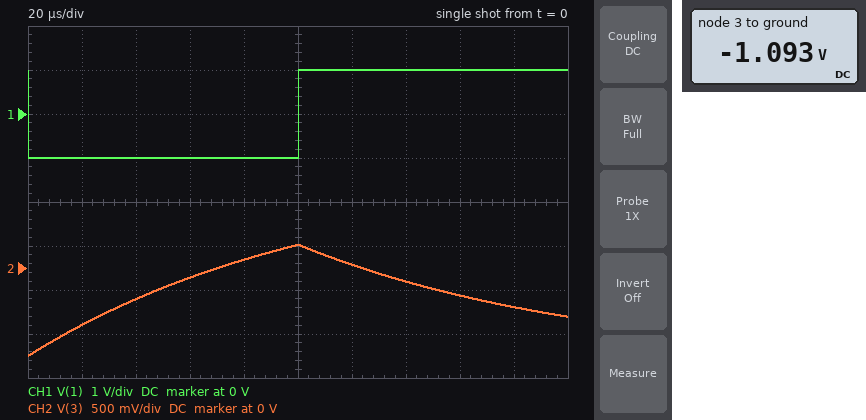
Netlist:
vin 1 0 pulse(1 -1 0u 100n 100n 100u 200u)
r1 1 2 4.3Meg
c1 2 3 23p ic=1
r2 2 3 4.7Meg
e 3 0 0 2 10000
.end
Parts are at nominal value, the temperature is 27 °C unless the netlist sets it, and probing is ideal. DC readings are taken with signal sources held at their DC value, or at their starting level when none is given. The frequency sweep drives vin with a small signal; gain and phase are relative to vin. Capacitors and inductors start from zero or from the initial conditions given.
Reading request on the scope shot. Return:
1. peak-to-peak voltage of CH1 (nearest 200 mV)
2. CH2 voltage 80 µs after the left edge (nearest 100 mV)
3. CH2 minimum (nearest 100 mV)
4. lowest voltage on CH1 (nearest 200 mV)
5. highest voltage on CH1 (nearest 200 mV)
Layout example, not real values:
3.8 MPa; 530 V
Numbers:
2.0 V; 100 mV; -1.0 V; -1.0 V; 1.0 V
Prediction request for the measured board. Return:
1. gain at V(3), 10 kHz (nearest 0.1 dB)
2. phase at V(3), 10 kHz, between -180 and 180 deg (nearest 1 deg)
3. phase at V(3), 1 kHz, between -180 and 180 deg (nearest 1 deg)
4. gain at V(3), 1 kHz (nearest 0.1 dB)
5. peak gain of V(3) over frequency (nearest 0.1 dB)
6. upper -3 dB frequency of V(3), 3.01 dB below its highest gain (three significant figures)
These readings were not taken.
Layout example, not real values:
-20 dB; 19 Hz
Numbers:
-16.0 dB; 98 deg; 146 deg; -0.9 dB; 0.8 dB; 1.47 kHz
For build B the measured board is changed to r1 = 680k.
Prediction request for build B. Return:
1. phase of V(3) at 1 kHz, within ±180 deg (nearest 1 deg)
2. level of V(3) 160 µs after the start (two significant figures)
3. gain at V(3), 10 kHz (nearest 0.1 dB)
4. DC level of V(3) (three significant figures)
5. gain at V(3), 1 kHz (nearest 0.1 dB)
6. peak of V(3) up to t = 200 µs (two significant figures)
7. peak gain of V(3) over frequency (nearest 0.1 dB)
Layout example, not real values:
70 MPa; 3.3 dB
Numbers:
146 deg; -770 mV; 0.1 dB; -6.91 V; 15.1 dB; 3.8 V; 16.8 dB
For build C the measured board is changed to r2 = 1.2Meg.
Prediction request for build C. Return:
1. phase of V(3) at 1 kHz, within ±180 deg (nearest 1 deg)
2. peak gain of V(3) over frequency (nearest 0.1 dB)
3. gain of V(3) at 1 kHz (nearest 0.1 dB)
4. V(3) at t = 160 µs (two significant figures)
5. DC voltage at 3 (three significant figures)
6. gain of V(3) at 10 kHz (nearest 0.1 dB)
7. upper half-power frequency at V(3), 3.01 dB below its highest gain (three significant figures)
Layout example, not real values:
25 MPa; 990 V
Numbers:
170 deg; -11.1 dB; -11.2 dB; -220 mV; -279 mV; -17.1 dB; 5.77 kHz
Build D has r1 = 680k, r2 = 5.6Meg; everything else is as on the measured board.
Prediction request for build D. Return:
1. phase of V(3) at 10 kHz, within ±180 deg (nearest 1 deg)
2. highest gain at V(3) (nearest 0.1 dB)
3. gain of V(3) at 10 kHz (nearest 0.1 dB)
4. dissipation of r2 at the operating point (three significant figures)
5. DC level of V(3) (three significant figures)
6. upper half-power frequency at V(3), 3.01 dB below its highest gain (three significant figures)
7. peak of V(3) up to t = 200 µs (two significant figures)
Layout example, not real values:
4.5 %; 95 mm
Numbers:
97 deg; 18.3 dB; 0.1 dB; 12.1 µW; -8.23 V; 1.24 kHz; 4.0 V
